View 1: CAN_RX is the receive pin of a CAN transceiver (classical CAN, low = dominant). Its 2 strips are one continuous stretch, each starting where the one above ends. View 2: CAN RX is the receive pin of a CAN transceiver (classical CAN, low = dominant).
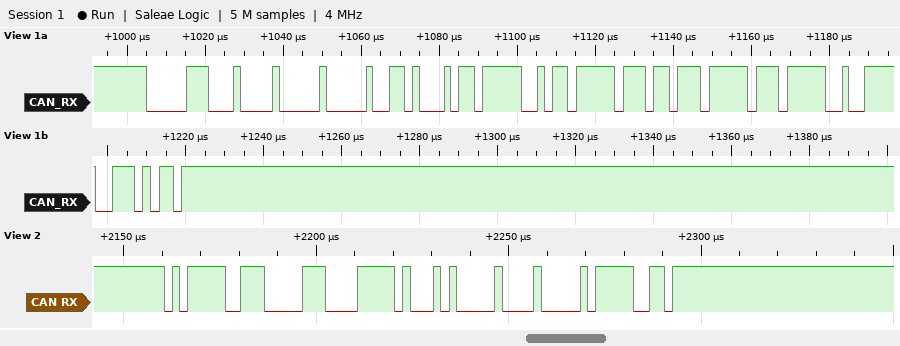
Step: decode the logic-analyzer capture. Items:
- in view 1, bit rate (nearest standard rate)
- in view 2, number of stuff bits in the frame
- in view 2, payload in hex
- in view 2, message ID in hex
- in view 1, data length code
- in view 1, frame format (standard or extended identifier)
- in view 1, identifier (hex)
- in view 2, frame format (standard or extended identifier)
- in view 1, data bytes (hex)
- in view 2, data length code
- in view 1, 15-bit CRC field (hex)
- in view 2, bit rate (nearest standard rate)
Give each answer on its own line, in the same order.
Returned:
500 kbit/s
6
0F C5 00
0x5F7
8
standard
0x062
standard
00 68 B7 D6 FF 6E FF 7D
3
0x1E75
500 kbit/s
